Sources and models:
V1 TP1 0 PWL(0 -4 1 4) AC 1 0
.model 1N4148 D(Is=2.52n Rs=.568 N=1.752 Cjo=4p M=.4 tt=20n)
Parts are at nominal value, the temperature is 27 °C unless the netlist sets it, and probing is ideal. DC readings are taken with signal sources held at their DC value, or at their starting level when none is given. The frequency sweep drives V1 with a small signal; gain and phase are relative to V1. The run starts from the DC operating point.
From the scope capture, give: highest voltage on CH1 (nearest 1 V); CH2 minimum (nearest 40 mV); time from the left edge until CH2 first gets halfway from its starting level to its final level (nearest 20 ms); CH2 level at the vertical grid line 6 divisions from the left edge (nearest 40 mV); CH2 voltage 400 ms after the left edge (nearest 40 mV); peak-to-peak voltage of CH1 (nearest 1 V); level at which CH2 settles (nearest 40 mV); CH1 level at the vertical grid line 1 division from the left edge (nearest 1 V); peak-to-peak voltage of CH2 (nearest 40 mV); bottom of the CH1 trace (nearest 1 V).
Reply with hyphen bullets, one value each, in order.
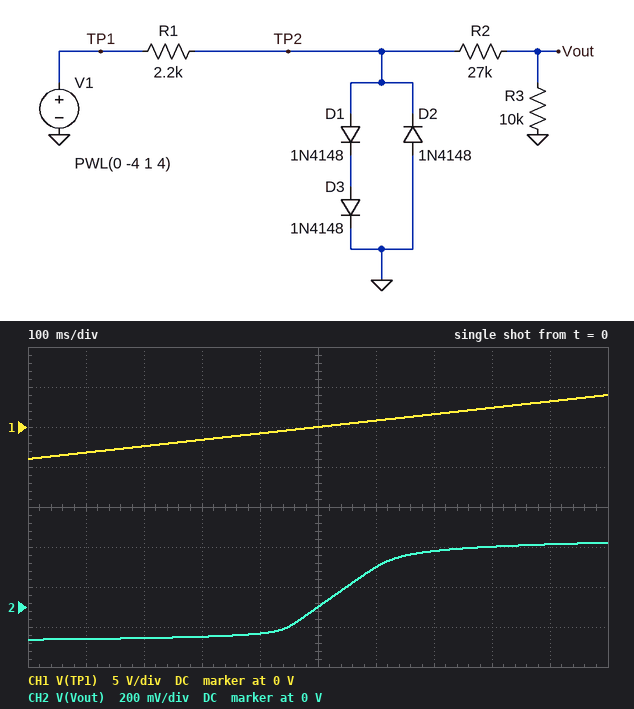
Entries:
- 4 V
- -160 mV
- 540 ms
- 200 mV
- -120 mV
- 8 V
- 320 mV
- -3 V
- 480 mV
- -4 V
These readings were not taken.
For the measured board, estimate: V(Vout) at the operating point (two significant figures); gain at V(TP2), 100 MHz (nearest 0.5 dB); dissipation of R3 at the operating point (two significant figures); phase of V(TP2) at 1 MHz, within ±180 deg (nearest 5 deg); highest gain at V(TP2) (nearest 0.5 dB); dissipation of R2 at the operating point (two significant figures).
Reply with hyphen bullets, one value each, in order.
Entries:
- -160 mV
- -59.0 dB
- 2.7 µW
- -5 deg
- -37.5 dB
- 7.2 µW
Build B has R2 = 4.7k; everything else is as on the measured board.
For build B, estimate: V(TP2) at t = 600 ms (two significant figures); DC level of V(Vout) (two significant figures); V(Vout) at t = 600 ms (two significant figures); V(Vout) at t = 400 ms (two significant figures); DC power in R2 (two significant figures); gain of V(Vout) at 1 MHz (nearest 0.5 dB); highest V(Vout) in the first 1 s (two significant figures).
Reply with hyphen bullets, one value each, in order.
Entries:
- 690 mV
- -410 mV
- 470 mV
- -330 mV
- 7.9 µW
- -40.5 dB
- 810 mV
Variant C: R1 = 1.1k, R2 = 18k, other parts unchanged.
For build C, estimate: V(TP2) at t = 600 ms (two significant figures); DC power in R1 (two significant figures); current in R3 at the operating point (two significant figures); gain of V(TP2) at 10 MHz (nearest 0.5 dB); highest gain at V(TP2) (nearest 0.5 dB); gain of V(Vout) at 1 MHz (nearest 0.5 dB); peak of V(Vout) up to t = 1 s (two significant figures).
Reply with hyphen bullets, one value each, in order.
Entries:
- 760 mV
- 10 mW
- 23 µA
- -41.0 dB
- -37.0 dB
- -46.0 dB
- 450 mV
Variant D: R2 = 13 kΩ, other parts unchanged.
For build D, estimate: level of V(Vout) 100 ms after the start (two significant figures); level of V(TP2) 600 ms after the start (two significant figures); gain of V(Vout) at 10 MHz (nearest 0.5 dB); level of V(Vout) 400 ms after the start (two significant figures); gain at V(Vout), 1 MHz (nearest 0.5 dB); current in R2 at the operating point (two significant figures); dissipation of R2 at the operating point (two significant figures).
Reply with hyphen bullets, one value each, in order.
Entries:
- -260 mV
- 720 mV
- -48.5 dB
- -210 mV
- -44.5 dB
- 26 µA
- 9.0 µW
